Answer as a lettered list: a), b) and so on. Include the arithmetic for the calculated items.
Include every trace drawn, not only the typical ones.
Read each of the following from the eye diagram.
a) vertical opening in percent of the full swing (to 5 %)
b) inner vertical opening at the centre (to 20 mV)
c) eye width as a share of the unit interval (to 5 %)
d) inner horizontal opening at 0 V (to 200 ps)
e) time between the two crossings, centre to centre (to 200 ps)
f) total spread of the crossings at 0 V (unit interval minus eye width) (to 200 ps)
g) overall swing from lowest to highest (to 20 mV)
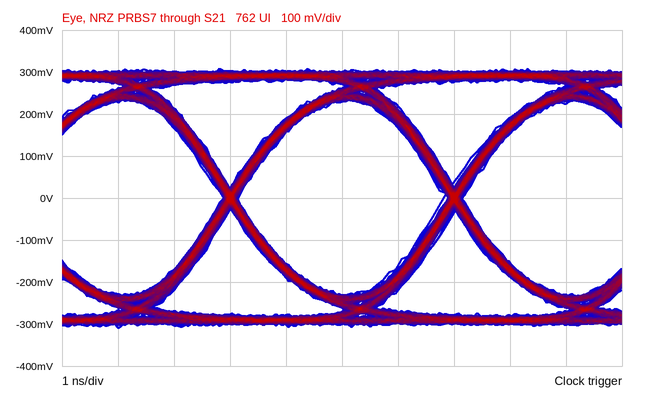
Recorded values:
a) 460 mV / 620 mV ≈ 74.2 %, so 75 % to the nearest 5 %
b) 460 mV
c) 3.6 ns / 4.0 ns ≈ 90 %
d) 3.6 ns
e) 4.0 ns
f) 400 ps
g) 620 mV
